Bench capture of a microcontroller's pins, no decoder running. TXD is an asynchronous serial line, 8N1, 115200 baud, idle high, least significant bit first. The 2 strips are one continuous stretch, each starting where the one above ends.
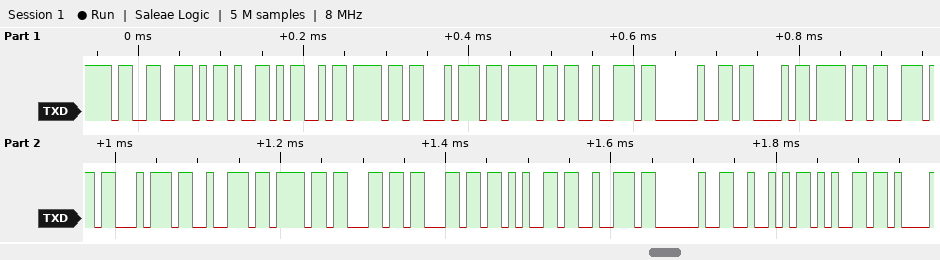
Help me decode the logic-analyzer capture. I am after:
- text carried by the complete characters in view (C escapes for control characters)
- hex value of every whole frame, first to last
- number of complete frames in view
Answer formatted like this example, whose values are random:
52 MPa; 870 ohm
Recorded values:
"3-Motor Controller Re"; 33 2D 4D 6F 74 6F 72 20 43 6F 6E 74 72 6F 6C 6C 65 72 20 52 65; 21
